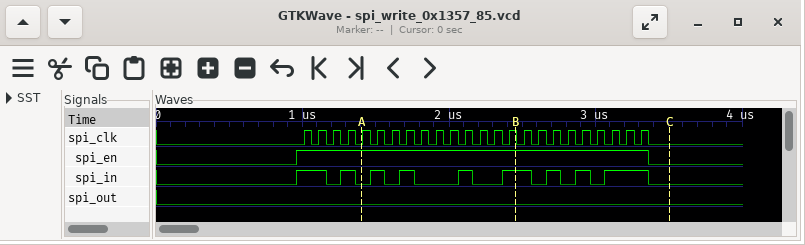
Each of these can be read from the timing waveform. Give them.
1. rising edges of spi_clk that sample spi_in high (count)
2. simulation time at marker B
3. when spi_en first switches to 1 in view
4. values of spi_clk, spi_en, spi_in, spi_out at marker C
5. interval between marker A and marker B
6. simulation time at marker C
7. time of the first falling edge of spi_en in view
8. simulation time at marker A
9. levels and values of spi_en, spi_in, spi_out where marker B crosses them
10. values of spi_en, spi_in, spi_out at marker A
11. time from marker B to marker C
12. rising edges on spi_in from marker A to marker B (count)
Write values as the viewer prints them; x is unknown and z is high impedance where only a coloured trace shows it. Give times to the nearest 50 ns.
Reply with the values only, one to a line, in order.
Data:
13
2450 ns
950 ns
spi_clk=0, spi_en=0, spi_in=0, spi_out=0
1050 ns
3500 ns
3350 ns
1400 ns
spi_en=1, spi_in=1, spi_out=0
spi_en=1, spi_in=0, spi_out=0
1050 ns
4
